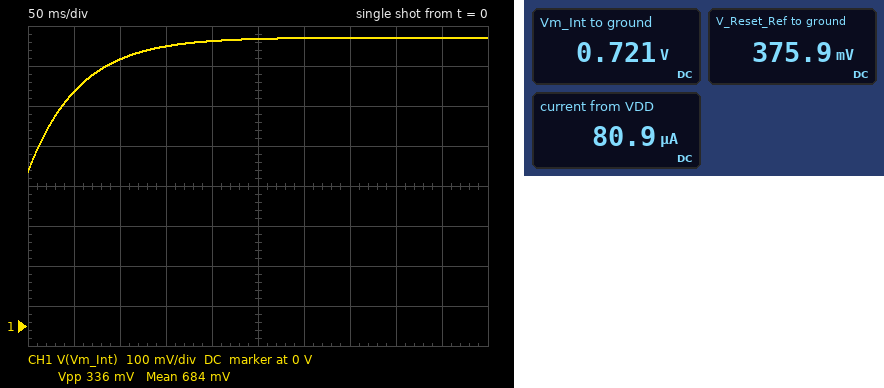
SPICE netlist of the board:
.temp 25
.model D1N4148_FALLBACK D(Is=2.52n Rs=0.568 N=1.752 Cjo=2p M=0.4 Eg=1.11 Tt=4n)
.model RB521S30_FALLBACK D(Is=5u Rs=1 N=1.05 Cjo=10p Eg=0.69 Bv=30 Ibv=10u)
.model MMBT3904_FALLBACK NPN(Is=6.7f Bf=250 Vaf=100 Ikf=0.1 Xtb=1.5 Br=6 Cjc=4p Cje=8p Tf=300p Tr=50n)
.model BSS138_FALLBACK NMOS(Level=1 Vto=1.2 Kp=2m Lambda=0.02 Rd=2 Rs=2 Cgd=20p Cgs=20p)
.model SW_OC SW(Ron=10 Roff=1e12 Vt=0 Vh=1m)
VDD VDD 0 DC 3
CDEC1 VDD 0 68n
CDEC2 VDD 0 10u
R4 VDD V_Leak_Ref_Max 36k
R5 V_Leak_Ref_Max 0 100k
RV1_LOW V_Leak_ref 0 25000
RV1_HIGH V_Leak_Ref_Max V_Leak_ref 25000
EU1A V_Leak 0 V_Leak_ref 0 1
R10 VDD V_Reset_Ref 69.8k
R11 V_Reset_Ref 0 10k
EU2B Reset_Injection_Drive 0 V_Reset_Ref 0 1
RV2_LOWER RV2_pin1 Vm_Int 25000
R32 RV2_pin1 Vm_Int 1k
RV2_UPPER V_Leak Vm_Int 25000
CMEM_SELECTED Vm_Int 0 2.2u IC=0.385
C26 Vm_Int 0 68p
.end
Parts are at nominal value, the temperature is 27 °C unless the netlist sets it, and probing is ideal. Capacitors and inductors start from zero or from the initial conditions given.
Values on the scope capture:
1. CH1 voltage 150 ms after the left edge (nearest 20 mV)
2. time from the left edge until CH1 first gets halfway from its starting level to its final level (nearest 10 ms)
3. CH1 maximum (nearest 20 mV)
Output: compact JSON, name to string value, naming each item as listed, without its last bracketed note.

{"CH1 voltage 150 ms after the left edge": "700 mV", "time from the left edge until CH1 first gets halfway from its starting level to its final level": "40 ms", "CH1 maximum": "720 mV"}
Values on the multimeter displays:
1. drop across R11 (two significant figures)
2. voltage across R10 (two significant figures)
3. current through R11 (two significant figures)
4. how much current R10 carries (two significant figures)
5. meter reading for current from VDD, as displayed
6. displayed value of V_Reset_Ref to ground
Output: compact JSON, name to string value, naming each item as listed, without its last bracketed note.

{"drop across R11": "380 mV", "voltage across R10": "2.6 V", "current through R11": "38 µA", "how much current R10 carries": "38 µA", "meter reading for current from VDD, as displayed": "80.9 µA", "displayed value of V_Reset_Ref to ground": "375.9 mV"}
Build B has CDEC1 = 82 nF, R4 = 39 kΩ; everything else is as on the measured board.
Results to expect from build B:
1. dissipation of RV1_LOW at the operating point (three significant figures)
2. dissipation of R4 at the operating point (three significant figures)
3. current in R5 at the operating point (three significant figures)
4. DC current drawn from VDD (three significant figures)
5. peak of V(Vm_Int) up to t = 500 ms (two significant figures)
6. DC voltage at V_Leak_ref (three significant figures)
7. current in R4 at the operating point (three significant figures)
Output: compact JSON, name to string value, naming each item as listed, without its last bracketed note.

{"dissipation of RV1_LOW at the operating point": "19.1 µW", "dissipation of R4 at the operating point": "67.1 µW", "current in R5 at the operating point": "13.8 µA", "DC current drawn from VDD": "79.1 µA", "peak of V(Vm_Int) up to t = 500 ms": "690 mV", "DC voltage at V_Leak_ref": "691 mV", "current in R4 at the operating point": "41.5 µA"}
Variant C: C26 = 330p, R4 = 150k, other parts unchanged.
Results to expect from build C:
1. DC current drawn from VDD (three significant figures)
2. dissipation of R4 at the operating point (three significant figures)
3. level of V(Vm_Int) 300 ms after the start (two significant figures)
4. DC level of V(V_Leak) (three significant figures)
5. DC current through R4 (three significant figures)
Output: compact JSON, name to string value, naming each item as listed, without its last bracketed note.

{"DC current drawn from VDD": "54.0 µA", "dissipation of R4 at the operating point": "40.2 µW", "level of V(Vm_Int) 300 ms after the start": "270 mV", "DC level of V(V_Leak)": "273 mV", "DC current through R4": "16.4 µA"}
